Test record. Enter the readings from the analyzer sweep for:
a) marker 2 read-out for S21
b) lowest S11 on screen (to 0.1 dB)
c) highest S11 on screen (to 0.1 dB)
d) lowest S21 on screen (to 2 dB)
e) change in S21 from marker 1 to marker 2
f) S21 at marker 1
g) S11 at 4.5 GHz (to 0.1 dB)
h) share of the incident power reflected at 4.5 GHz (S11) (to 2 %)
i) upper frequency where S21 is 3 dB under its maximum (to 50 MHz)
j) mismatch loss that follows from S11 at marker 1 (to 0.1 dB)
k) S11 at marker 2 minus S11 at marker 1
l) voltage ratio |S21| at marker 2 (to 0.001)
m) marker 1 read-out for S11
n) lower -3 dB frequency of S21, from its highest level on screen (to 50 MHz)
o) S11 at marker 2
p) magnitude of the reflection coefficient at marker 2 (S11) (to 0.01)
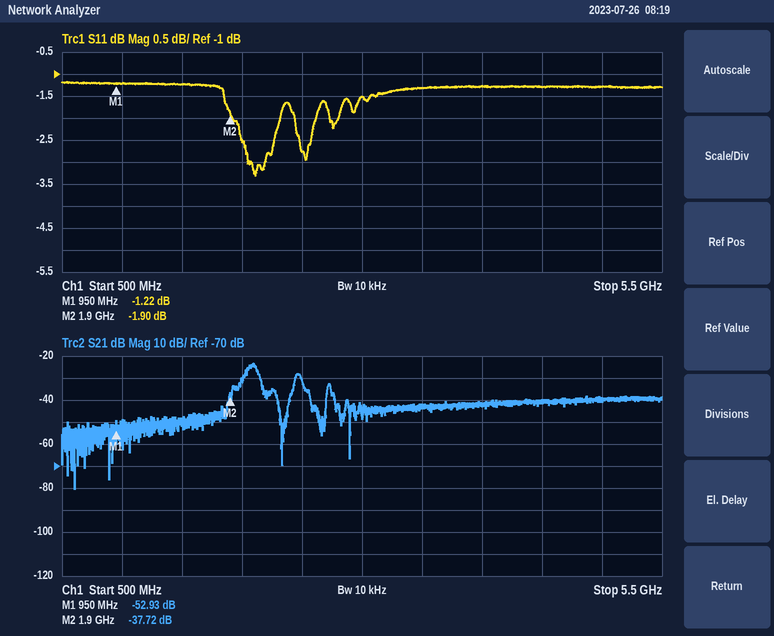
-37.72 dB
-3.3 dB
-1.2 dB
-80 dB
15.21 dB
-52.93 dB
-1.3 dB
74 %
2.10 GHz
6.1 dB
-0.68 dB
0.013
-1.22 dB
2.05 GHz
-1.90 dB
0.80
